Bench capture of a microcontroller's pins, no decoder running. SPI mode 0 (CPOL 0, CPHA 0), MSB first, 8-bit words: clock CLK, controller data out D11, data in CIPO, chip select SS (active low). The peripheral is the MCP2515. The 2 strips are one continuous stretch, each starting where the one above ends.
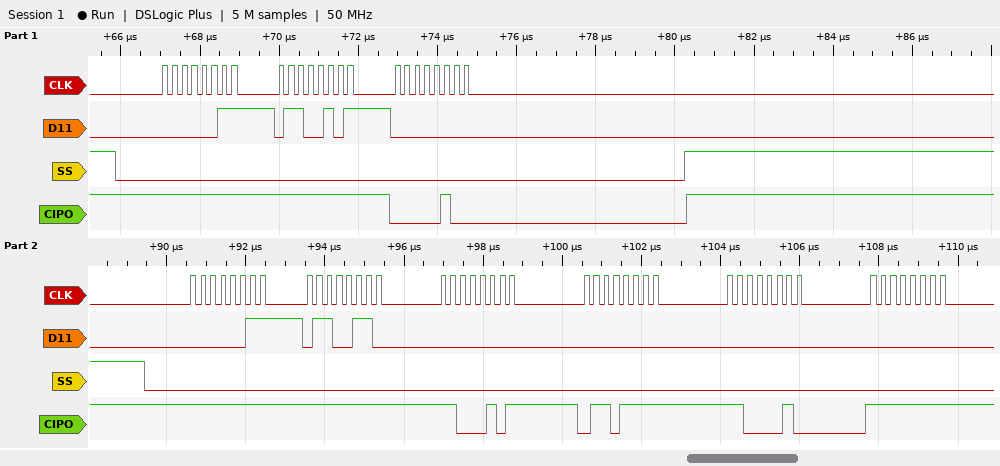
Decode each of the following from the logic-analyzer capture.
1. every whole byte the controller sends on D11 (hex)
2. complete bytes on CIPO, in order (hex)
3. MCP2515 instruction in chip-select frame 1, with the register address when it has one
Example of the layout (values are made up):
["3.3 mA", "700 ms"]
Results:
["03 65 00 03 66 00 00 00 00", "FF FF 04 FF FF C5 6F C2 FF", "READ 0x65"]
